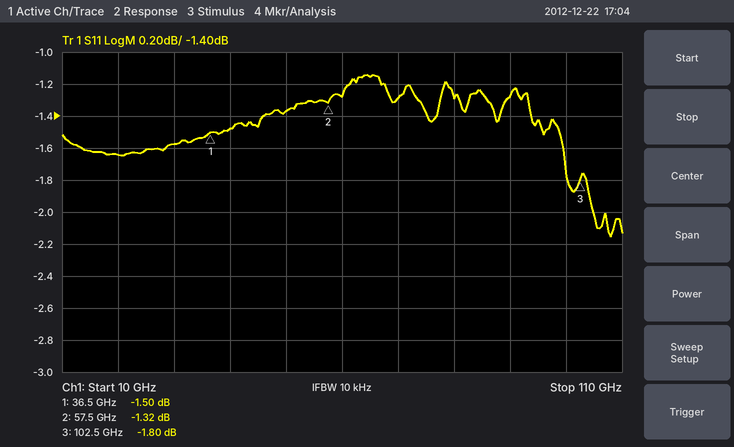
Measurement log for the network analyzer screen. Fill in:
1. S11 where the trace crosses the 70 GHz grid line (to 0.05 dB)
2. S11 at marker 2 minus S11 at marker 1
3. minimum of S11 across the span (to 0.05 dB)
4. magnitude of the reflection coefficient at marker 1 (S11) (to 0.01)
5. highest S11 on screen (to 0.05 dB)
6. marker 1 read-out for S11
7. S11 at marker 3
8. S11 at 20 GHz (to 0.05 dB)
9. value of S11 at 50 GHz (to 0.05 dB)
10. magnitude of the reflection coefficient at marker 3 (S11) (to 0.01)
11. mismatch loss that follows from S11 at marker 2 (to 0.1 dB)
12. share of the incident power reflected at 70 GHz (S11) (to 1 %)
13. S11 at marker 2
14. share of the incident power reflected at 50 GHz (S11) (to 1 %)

-1.30 dB
0.18 dB
-2.15 dB
0.84
-1.15 dB
-1.50 dB
-1.80 dB
-1.65 dB
-1.35 dB
0.81
5.8 dB
74 %
-1.32 dB
73 %
